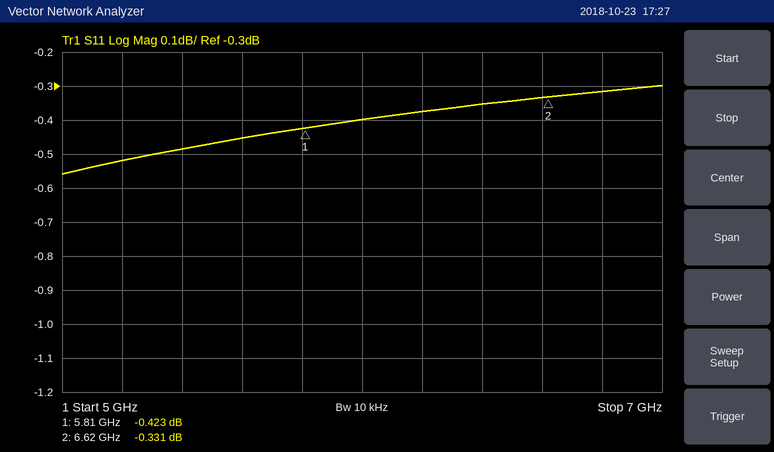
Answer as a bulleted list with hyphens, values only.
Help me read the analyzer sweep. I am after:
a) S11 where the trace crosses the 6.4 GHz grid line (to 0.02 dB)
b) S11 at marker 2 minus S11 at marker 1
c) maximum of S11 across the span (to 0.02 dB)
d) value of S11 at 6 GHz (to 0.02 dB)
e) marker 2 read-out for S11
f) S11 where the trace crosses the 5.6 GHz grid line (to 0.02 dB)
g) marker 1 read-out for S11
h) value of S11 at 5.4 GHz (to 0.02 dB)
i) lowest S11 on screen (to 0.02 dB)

- -0.36 dB
- 0.092 dB
- -0.30 dB
- -0.40 dB
- -0.331 dB
- -0.46 dB
- -0.423 dB
- -0.48 dB
- -0.56 dB
